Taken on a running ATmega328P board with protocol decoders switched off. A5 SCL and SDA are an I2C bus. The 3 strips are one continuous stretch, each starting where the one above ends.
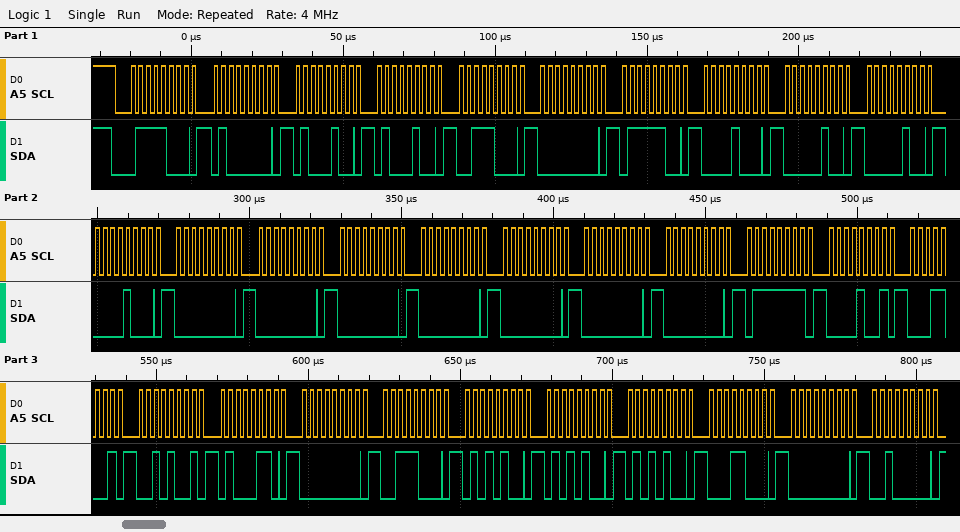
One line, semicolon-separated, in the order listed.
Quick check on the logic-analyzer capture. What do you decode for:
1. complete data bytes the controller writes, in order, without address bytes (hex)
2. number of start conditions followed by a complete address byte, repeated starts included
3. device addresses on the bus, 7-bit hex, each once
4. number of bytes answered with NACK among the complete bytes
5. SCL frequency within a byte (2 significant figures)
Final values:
40 44 44 38 00 7C 08 04 04 08 00 00 00 00 00 00 00 7F 09 19 29 46 00 38 54 54 54 18 00 20; 1; 0x3C; 0; 400 kHz
